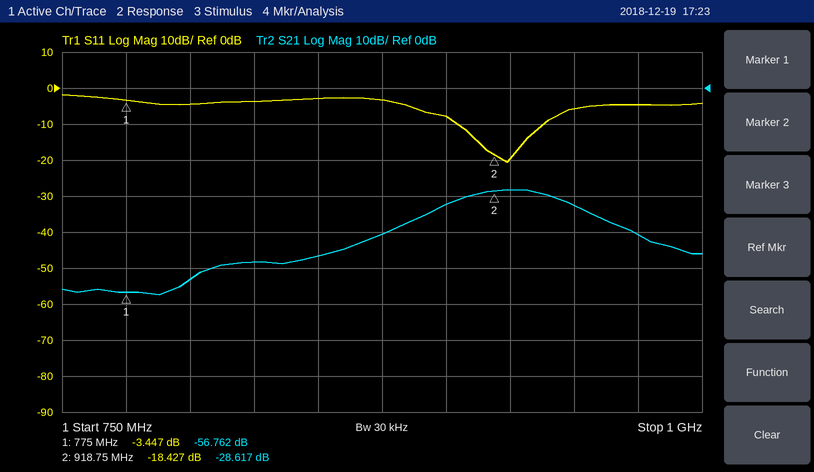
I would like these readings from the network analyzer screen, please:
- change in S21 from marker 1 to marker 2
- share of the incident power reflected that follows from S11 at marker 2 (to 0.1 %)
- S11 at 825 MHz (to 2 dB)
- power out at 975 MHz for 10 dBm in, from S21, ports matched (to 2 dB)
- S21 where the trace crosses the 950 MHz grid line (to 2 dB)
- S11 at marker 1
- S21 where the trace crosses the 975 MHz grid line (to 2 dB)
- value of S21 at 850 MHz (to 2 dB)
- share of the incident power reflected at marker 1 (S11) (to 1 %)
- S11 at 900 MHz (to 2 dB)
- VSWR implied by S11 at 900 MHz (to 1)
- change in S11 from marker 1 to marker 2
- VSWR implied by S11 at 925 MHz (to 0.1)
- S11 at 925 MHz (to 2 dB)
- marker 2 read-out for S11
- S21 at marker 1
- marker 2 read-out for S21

28.145 dB
1.4 %
-4 dB
-30 dBm
-32 dB
-3.447 dB
-40 dB
-46 dB
45 %
-8 dB
2
-14.980 dB
1.2
-20 dB
-18.427 dB
-56.762 dB
-28.617 dB
